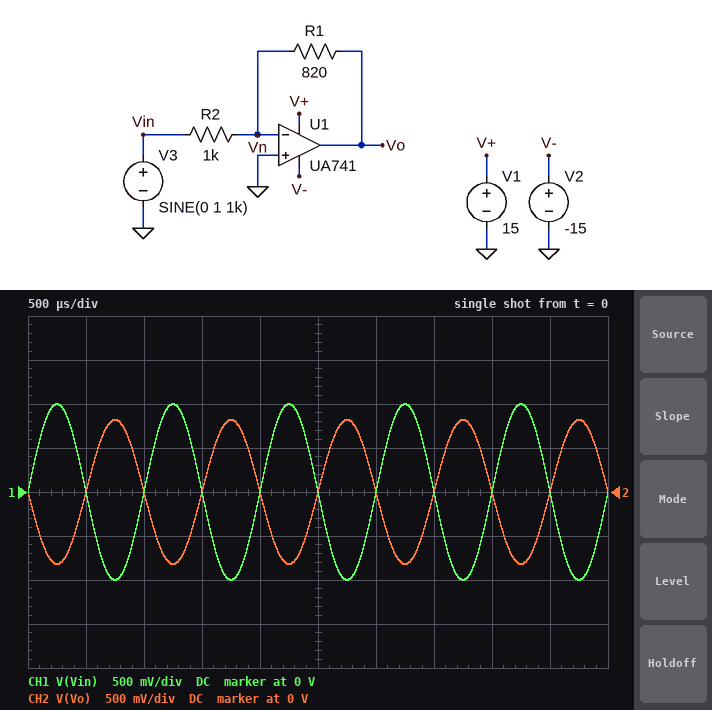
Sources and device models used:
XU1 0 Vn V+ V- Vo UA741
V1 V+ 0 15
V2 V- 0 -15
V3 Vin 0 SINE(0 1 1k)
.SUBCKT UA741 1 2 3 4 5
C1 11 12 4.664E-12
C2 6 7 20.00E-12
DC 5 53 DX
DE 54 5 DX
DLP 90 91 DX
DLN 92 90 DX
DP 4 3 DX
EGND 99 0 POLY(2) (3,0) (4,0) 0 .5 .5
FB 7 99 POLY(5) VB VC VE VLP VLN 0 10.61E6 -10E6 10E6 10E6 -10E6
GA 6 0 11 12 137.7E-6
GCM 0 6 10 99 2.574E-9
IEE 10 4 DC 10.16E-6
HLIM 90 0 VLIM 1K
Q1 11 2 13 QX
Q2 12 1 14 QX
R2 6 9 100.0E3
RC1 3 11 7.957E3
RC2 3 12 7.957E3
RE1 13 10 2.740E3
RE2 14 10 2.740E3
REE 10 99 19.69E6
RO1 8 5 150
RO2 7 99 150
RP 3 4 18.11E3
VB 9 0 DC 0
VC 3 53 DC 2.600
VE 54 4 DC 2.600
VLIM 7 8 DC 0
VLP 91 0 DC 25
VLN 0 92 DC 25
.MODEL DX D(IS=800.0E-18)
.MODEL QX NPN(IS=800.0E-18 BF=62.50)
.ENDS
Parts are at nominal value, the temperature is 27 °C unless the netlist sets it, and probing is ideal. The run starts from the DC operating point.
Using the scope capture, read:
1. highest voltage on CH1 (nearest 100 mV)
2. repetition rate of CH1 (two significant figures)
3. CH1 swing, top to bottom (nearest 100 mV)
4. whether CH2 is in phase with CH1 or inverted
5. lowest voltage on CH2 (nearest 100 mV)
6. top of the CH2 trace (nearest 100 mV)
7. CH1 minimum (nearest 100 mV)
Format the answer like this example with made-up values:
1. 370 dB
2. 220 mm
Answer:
1. 1.0 V
2. 1.0 kHz
3. 2.0 V
4. inverted
5. -800 mV
6. 800 mV
7. -1.0 V
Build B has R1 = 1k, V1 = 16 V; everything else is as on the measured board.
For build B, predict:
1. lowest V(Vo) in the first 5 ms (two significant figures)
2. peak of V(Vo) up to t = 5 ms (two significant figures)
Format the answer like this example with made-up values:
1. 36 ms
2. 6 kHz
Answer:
1. -1.0 V
2. 1.0 V
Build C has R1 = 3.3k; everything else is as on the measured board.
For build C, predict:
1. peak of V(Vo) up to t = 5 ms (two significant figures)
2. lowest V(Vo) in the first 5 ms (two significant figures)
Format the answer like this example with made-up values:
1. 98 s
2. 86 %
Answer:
1. 3.3 V
2. -3.3 V
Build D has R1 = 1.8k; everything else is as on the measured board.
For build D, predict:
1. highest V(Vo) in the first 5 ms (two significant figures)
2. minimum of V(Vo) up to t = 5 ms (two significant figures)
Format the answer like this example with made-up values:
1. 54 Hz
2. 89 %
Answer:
1. 1.8 V
2. -1.8 V
